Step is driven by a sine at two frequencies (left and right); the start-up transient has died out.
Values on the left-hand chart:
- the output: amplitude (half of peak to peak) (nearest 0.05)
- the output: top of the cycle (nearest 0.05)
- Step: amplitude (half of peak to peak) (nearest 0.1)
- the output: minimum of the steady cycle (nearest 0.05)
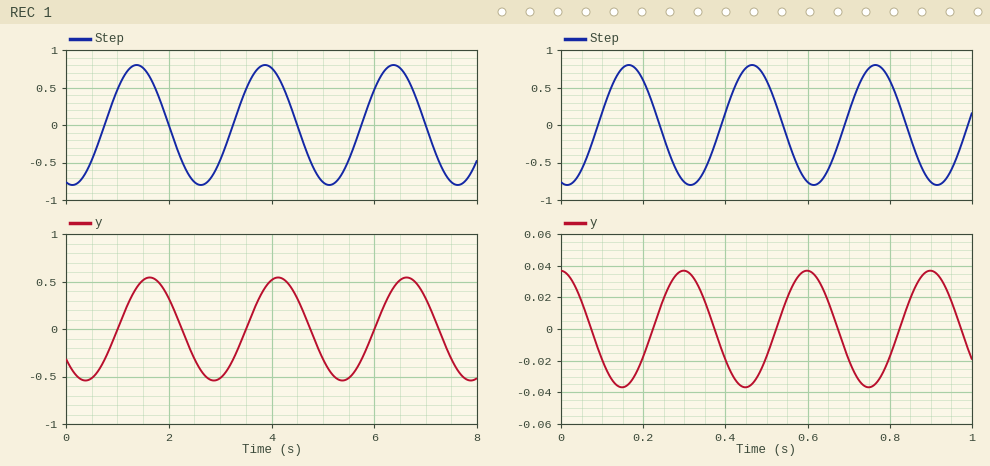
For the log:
0.55
0.55
0.8
-0.55
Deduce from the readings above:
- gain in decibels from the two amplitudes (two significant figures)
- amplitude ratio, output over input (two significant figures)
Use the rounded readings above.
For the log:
-3.3 dB
0.69
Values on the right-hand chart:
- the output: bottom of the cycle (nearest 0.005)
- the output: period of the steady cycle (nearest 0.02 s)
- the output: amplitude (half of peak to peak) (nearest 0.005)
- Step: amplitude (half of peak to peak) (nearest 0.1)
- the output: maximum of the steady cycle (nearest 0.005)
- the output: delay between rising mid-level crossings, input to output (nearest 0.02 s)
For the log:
-0.035
0.30 s
0.035
0.8
0.035
0.14 s
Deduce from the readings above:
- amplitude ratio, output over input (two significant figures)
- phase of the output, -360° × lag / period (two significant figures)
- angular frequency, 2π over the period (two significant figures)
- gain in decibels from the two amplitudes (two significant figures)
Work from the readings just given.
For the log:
0.044
-170°
21 rad/s
-27 dB
